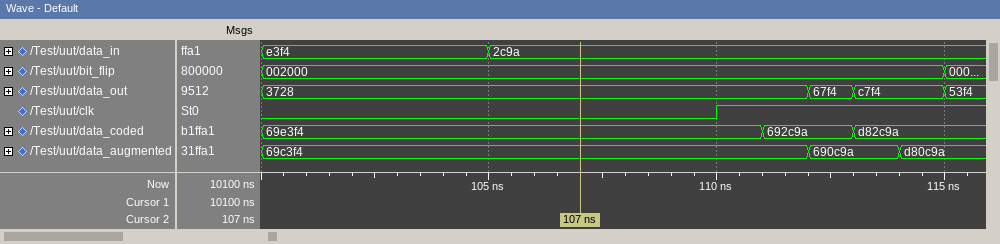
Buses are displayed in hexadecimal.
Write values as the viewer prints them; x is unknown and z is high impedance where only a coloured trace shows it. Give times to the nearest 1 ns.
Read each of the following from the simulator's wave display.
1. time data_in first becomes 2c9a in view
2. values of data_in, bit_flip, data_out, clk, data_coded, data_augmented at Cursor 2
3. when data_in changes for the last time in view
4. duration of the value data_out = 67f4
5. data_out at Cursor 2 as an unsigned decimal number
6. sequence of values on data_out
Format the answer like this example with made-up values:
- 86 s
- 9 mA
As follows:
- 105 ns
- data_in=2c9a, bit_flip=002000, data_out=3728, clk=0, data_coded=69e3f4, data_augmented=69c3f4
- 105 ns
- 1 ns
- 14120
- 3728, 67f4, c7f4, 53f4
